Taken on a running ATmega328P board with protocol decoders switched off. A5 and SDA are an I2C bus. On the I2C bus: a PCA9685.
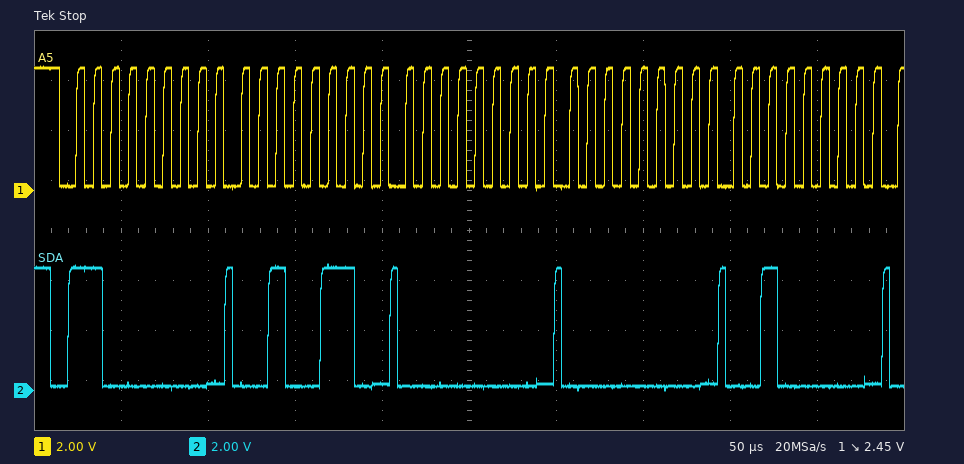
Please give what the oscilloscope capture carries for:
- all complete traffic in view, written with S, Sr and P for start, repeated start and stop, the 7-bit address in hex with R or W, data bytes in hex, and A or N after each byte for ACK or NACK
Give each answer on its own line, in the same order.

S 60W A 26 A 00 A 00 A 20 A
